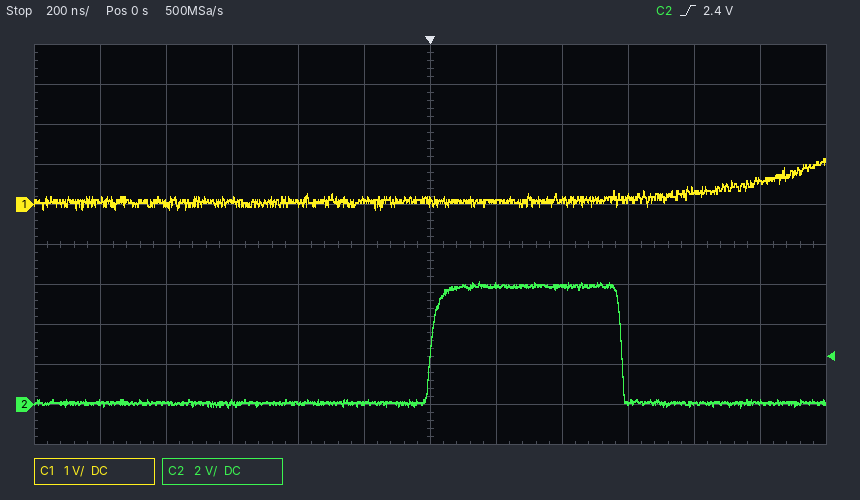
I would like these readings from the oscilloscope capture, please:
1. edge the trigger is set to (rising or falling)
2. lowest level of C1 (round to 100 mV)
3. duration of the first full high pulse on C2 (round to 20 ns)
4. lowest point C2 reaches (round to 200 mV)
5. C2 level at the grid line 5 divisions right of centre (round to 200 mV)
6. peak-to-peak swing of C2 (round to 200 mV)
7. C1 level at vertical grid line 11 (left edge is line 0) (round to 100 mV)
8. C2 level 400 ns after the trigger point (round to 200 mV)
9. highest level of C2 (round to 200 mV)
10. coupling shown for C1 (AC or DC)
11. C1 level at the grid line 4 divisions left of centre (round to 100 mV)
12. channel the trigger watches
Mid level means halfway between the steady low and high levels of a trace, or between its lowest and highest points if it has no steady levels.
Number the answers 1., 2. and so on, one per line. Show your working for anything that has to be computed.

1. rising
2. -100 mV
3. 580 ns
4. -200 mV
5. 200 mV
6. 6.2 V − (-200 mV) = 6.4 V
7. 600 mV
8. 6.0 V
9. 6.2 V
10. DC
11. 0.0 V
12. C2
